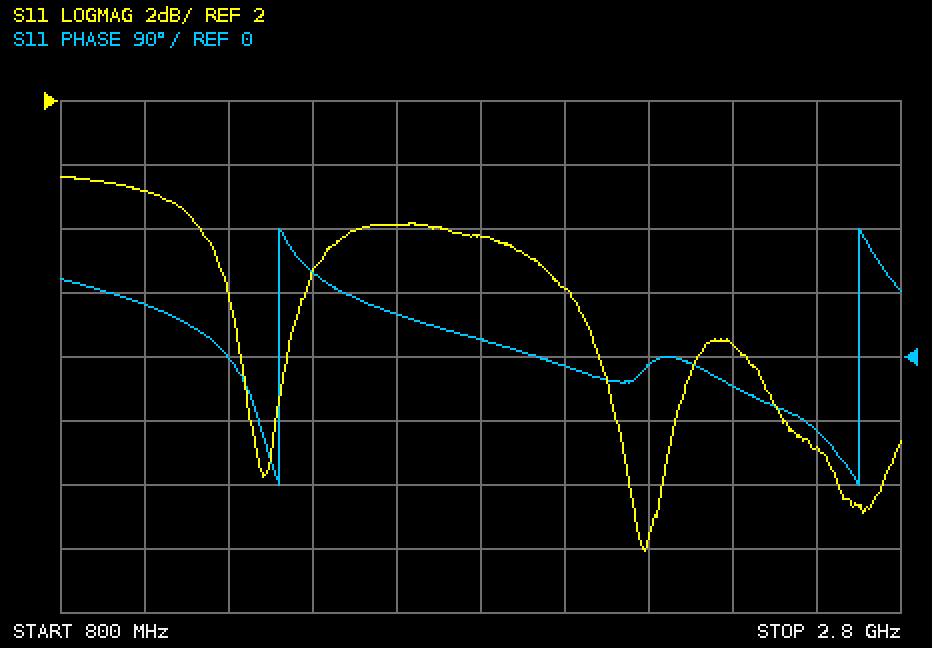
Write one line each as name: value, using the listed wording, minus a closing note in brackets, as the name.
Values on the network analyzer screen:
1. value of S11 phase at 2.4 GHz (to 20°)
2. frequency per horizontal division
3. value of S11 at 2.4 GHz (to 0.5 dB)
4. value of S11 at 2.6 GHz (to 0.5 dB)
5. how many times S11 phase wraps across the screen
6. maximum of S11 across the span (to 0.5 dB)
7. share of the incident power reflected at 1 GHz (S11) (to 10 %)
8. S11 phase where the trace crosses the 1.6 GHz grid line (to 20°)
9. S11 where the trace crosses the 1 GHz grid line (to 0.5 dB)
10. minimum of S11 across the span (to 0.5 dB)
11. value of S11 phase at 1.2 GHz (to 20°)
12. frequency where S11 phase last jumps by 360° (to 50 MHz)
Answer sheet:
value of S11 phase at 2.4 GHz: -40°
frequency per horizontal division: 200 MHz
value of S11 at 2.4 GHz: -5.5 dB
value of S11 at 2.6 GHz: -9.0 dB
how many times S11 phase wraps across the screen: 2
maximum of S11 across the span: -0.5 dB
share of the incident power reflected at 1 GHz (S11): 80 %
S11 phase where the trace crosses the 1.6 GHz grid line: 60°
S11 where the trace crosses the 1 GHz grid line: -1.0 dB
minimum of S11 across the span: -12.0 dB
value of S11 phase at 1.2 GHz: 0°
frequency where S11 phase last jumps by 360°: 2.70 GHz
